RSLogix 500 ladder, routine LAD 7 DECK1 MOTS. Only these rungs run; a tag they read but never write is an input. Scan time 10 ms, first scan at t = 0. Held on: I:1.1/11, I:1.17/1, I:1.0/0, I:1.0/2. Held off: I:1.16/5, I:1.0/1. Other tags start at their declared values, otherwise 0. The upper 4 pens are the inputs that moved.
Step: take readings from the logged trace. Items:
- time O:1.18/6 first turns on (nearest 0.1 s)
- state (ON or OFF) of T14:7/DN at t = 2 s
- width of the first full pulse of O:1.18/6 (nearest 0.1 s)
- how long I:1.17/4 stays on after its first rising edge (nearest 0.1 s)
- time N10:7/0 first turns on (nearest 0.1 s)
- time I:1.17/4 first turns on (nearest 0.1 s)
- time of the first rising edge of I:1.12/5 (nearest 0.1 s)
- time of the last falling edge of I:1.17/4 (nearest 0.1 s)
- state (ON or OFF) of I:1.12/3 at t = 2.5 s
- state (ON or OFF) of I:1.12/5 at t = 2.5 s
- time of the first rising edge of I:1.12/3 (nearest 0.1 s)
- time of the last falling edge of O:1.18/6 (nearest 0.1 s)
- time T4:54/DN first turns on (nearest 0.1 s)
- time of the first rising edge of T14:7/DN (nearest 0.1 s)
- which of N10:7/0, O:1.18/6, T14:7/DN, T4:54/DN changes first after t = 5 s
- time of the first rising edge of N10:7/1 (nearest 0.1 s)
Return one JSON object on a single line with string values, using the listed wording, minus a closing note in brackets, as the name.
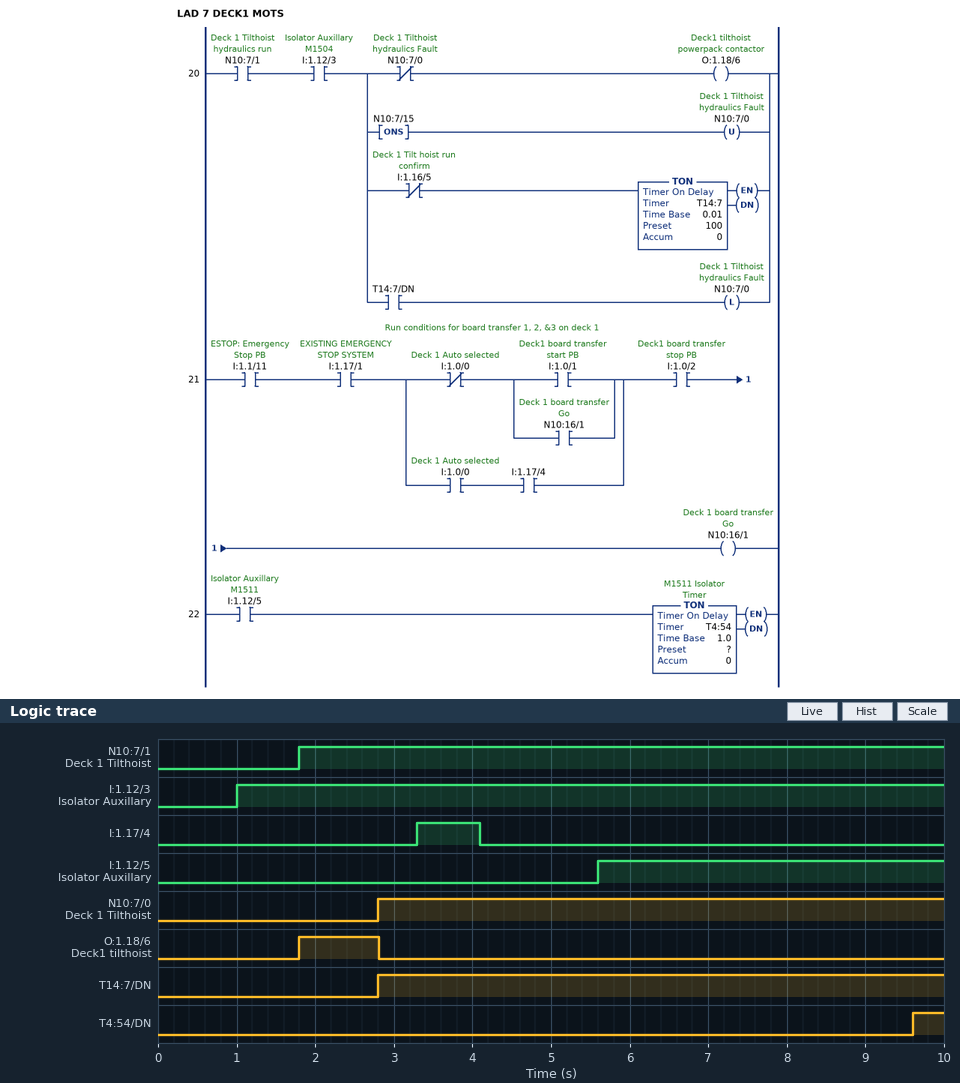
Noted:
{"time O:1.18/6 first turns on": "1.8 s", "state (ON or OFF) of T14:7/DN at t = 2 s": "OFF", "width of the first full pulse of O:1.18/6": "1.0 s", "how long I:1.17/4 stays on after its first rising edge": "0.8 s", "time N10:7/0 first turns on": "2.8 s", "time I:1.17/4 first turns on": "3.3 s", "time of the first rising edge of I:1.12/5": "5.6 s", "time of the last falling edge of I:1.17/4": "4.1 s", "state (ON or OFF) of I:1.12/3 at t = 2.5 s": "ON", "state (ON or OFF) of I:1.12/5 at t = 2.5 s": "OFF", "time of the first rising edge of I:1.12/3": "1.0 s", "time of the last falling edge of O:1.18/6": "2.8 s", "time T4:54/DN first turns on": "9.6 s", "time of the first rising edge of T14:7/DN": "2.8 s", "which of N10:7/0, O:1.18/6, T14:7/DN, T4:54/DN changes first after t = 5 s": "T4:54/DN", "time of the first rising edge of N10:7/1": "1.8 s"}
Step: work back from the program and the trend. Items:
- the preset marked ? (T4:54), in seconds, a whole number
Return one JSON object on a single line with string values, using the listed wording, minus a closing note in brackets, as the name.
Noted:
{"the preset marked ? (T4:54), in seconds, a whole number": "4 s"}
